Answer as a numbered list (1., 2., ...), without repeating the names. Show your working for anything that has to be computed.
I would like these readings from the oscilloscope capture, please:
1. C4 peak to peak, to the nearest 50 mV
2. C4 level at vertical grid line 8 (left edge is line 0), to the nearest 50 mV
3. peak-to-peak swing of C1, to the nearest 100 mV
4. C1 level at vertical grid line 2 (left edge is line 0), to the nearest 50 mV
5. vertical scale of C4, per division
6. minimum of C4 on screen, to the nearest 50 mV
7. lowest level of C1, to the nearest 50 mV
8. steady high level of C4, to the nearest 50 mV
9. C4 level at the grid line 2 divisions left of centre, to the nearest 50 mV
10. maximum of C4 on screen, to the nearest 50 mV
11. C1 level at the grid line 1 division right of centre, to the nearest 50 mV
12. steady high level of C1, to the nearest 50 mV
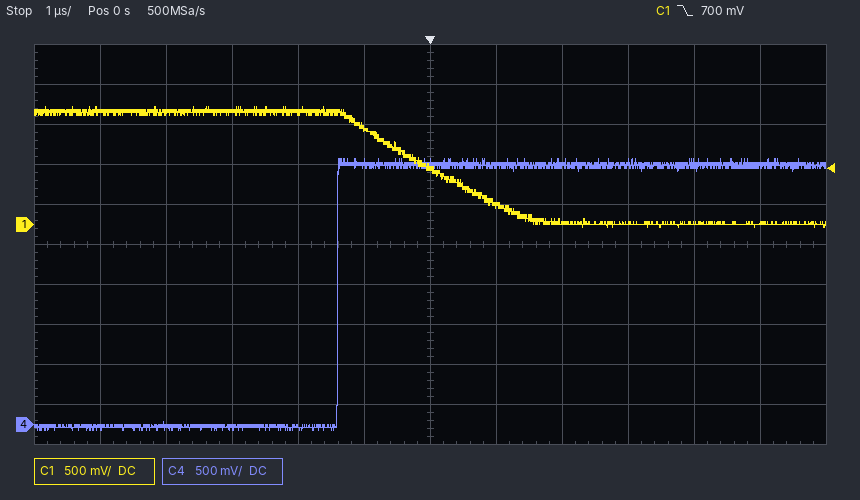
1. 3.30 V − (-100 mV) = 3.40 V
2. 3.25 V
3. 1.50 V
4. 1.40 V
5. 500 mV
6. -100 mV
7. -50 mV
8. 3.25 V
9. -50 mV
10. 3.30 V
11. 250 mV
12. 1.40 V
